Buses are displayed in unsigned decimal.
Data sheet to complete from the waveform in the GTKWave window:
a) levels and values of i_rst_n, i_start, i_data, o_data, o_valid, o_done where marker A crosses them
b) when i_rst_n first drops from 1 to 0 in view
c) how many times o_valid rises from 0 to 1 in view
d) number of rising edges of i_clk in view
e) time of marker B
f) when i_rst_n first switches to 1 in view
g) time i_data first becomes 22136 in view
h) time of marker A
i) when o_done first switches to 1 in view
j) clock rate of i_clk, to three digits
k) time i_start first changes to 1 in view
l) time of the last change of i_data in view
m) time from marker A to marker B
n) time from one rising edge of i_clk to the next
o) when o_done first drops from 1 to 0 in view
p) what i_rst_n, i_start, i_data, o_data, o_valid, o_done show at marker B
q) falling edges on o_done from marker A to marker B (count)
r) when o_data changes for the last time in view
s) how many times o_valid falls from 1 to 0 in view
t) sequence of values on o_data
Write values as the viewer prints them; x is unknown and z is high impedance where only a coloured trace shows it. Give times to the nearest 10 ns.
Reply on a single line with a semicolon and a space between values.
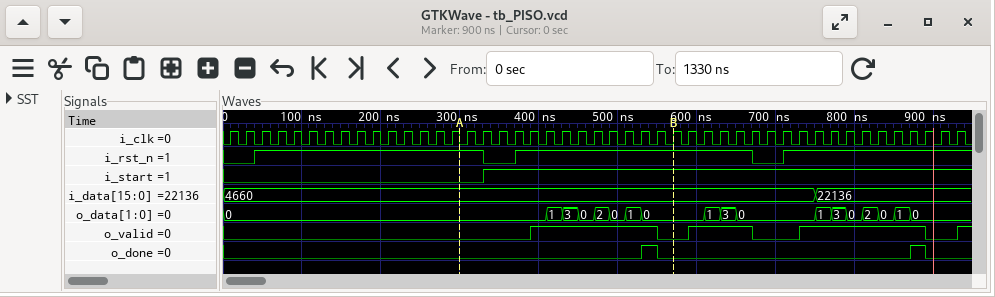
i_rst_n=1, i_start=0, i_data=4660, o_data=0, o_valid=0, o_done=0; 330 ns; 4; 47; 570 ns; 40 ns; 750 ns; 300 ns; 530 ns; 50.0 MHz; 330 ns; 750 ns; 270 ns; 20 ns; 550 ns; i_rst_n=1, i_start=1, i_data=4660, o_data=0, o_valid=0, o_done=0; 1; 870 ns; 3; 0, 1, 3, 0, 2, 0, 1, 0, 1, 3, 0, 1, 3, 0, 2, 0, 1, 0
